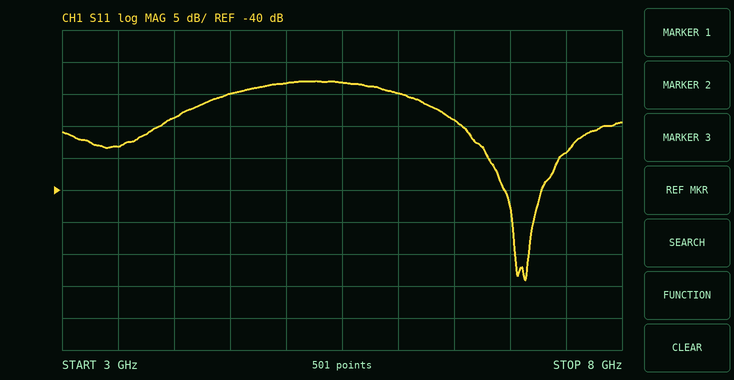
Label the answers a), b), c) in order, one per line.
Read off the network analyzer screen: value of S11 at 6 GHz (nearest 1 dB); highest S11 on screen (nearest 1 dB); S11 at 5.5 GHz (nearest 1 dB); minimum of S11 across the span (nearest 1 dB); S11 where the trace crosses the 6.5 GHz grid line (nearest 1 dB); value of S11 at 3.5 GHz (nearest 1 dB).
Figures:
a) -25 dB
b) -23 dB
c) -23 dB
d) -54 dB
e) -29 dB
f) -33 dB
